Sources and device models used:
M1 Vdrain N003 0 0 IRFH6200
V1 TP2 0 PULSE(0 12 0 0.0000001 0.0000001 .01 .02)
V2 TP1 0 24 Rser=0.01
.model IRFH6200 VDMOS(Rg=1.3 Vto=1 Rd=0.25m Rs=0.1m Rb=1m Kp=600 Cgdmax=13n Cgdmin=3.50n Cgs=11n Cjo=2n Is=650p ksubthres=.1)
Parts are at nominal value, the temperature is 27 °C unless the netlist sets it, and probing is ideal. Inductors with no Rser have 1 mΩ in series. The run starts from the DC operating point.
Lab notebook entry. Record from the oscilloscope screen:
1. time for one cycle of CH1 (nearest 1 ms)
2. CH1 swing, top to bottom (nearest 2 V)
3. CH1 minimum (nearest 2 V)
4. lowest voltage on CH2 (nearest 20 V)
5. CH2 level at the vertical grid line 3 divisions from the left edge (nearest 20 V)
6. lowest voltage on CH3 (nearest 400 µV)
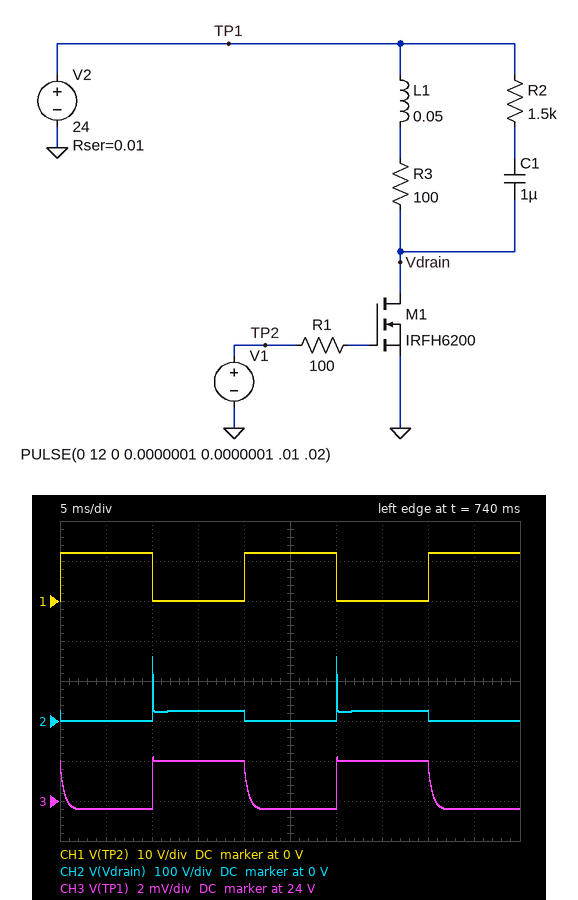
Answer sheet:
20 ms
12 V
0 V
0 V
20 V
23.9976 V
